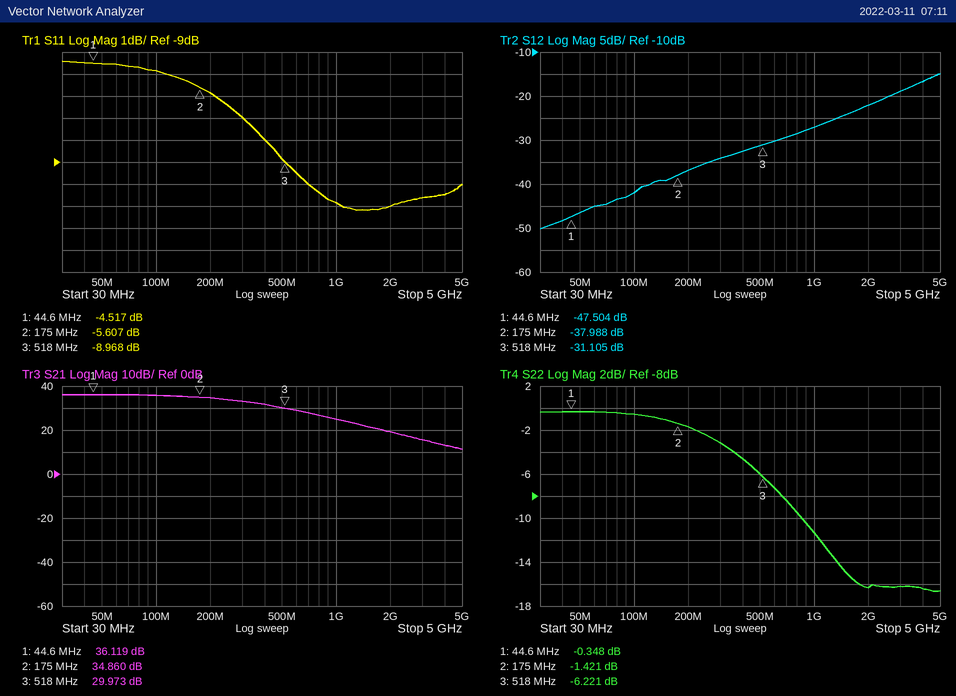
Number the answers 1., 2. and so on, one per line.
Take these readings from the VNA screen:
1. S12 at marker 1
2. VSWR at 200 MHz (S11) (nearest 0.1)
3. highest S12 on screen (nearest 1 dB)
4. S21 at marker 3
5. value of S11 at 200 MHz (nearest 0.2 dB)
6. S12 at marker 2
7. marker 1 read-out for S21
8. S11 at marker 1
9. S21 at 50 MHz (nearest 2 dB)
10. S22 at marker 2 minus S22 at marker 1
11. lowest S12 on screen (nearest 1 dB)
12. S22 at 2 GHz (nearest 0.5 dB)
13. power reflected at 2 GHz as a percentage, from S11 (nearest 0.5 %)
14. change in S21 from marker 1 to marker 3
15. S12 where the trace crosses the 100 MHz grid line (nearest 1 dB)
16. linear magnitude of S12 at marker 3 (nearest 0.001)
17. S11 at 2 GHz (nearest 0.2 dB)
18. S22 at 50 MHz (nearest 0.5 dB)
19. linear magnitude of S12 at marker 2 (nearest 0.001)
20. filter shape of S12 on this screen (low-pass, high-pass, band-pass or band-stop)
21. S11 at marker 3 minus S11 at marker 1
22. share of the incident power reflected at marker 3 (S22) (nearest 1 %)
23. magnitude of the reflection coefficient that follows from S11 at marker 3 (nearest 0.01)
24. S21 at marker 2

1. -47.504 dB
2. 3.1
3. -15 dB
4. 29.973 dB
5. -5.8 dB
6. -37.988 dB
7. 36.119 dB
8. -4.517 dB
9. 36 dB
10. -1.073 dB
11. -50 dB
12. -16.5 dB
13. 8.0 %
14. -6.146 dB
15. -42 dB
16. 0.028
17. -11.0 dB
18. -0.5 dB
19. 0.013
20. high-pass
21. -4.451 dB
22. 24 %
23. 0.36
24. 34.860 dB
